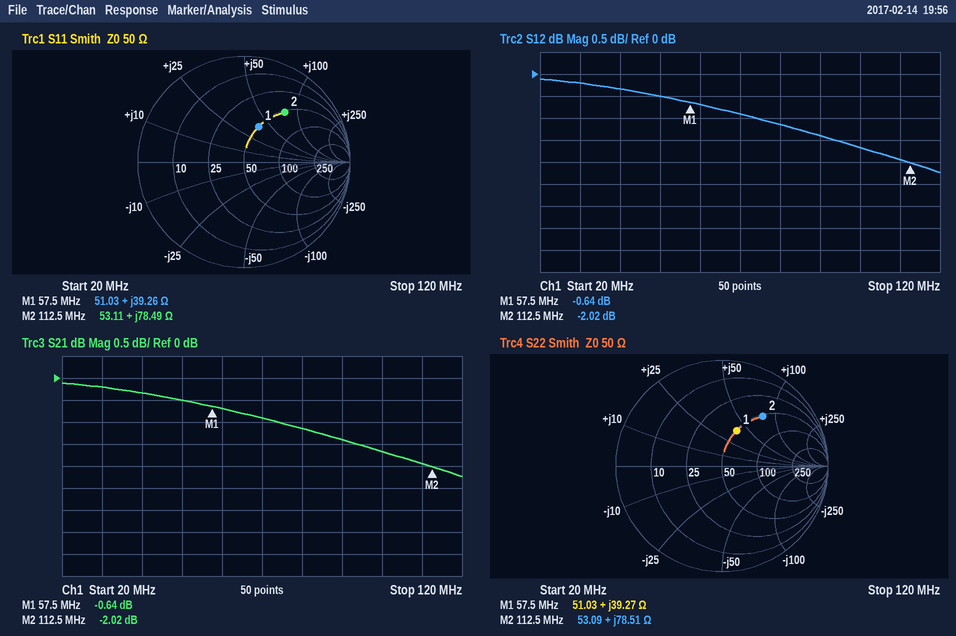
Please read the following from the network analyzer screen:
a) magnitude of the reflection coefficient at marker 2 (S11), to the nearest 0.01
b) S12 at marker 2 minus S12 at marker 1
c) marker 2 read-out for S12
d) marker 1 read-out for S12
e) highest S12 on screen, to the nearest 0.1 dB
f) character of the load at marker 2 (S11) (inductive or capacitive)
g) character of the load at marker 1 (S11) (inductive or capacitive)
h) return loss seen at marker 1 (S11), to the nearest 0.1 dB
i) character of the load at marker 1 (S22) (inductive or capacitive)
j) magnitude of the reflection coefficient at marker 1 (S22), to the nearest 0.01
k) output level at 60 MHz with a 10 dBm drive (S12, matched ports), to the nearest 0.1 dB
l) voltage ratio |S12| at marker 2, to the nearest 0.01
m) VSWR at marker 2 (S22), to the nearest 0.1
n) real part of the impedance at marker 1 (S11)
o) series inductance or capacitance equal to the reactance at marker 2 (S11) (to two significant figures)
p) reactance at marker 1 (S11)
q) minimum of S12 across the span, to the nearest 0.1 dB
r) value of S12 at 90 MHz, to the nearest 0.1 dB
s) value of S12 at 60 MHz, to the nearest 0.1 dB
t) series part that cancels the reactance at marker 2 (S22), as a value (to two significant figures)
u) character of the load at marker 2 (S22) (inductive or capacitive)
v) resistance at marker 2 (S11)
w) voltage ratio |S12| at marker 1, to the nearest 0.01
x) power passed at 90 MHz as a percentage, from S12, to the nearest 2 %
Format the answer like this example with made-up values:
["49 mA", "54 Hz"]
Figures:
["0.61", "-1.38 dB", "-2.02 dB", "-0.64 dB", "-0.1 dB", "inductive", "inductive", "8.8 dB", "inductive", "0.36", "9.3 dBm", "0.79", "4.1", "51.03 Ω", "110 nH", "+39.26 Ω", "-2.2 dB", "-1.4 dB", "-0.7 dB", "18 pF", "inductive", "53.11 Ω", "0.93", "72 %"]
